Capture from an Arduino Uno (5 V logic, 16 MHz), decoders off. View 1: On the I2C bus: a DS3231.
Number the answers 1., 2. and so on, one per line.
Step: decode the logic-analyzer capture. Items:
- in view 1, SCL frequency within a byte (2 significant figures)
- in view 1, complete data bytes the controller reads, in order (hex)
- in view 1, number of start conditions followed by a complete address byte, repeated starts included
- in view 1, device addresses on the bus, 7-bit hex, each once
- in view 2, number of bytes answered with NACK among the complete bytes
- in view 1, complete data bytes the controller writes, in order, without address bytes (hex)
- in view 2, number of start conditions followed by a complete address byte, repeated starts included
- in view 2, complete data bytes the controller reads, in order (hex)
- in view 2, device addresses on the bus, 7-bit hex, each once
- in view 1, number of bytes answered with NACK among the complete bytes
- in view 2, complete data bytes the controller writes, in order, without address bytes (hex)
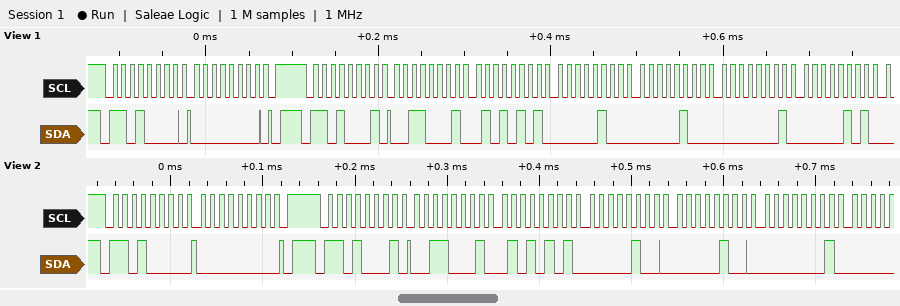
1. 100 kHz
2. 31 55 04 04 01 05
3. 2
4. 0x68
5. 0
6. 00
7. 2
8. 31 55 04 04 01
9. 0x68
10. 0
11. 00
